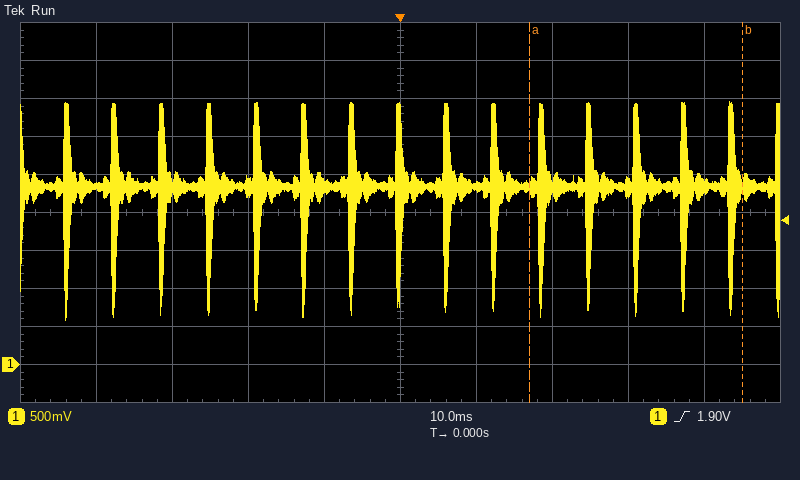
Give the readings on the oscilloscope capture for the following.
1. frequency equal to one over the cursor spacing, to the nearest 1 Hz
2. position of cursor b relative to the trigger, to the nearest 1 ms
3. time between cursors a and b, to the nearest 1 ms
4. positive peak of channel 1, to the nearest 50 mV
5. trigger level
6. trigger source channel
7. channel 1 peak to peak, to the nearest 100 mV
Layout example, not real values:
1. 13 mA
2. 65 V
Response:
1. 36 Hz
2. +45 ms
3. 28 ms
4. 3.45 V
5. 1.90 V
6. channel 1
7. 2.90 V
